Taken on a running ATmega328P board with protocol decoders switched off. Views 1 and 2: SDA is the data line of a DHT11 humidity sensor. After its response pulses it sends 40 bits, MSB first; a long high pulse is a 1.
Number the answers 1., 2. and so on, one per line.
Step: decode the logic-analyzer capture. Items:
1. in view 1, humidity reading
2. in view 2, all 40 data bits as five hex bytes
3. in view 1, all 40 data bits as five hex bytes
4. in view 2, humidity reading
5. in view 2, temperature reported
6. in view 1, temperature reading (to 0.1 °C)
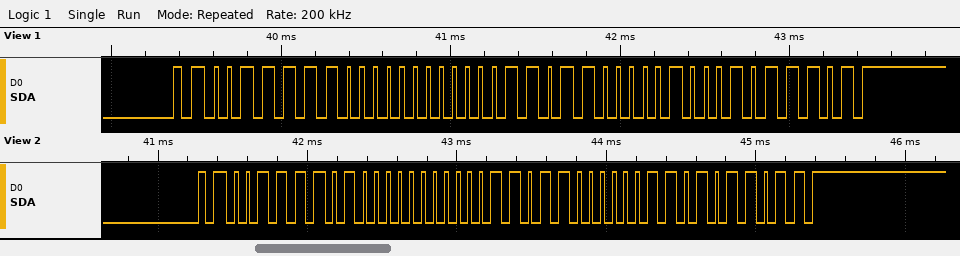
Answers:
1. 62 %
2. 3D 00 1B 03 5B
3. 3E 00 1B 04 5D
4. 61 %
5. 27.3 °C
6. 27.4 °C
